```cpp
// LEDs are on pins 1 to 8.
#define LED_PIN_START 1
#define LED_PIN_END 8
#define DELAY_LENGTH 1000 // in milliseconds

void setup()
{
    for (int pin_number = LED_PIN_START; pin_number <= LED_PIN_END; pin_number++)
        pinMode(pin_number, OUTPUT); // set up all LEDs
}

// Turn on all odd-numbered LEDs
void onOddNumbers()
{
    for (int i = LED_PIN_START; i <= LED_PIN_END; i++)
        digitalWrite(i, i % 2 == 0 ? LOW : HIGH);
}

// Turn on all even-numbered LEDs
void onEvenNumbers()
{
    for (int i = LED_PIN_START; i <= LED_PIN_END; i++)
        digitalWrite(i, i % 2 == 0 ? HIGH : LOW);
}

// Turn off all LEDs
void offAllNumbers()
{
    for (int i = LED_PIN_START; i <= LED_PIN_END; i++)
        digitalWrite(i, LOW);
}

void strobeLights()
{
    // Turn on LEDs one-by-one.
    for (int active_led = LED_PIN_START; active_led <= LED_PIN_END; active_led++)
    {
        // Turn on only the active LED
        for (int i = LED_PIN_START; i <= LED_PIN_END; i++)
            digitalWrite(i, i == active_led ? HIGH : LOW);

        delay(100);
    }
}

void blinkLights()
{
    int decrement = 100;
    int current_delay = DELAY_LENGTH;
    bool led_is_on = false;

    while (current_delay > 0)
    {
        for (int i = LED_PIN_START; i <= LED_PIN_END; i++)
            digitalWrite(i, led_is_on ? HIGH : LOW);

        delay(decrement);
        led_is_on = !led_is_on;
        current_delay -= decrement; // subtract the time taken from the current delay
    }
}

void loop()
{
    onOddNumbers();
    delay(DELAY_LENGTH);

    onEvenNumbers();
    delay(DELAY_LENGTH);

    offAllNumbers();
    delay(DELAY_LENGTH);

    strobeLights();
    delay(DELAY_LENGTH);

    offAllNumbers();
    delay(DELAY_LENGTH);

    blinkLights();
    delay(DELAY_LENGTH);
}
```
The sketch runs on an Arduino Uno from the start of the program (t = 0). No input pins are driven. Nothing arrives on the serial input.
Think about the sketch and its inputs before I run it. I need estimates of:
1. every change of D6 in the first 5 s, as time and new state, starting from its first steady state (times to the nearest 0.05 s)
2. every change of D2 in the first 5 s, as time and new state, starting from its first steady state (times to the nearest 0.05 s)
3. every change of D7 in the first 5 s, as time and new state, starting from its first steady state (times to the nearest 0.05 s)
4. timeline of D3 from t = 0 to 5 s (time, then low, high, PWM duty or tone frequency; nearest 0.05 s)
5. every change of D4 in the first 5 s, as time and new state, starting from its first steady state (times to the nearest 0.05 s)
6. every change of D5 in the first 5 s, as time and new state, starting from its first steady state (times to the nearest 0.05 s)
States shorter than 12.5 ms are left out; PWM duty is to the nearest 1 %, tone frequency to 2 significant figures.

0 s low; 1 s high; 2 s low; 3.5 s high; 3.6 s low
0 s low; 1 s high; 2 s low; 3.1 s high; 3.2 s low
0 s high; 1 s low; 3.6 s high; 3.7 s low
0 s high; 1 s low; 3.2 s high; 3.3 s low
0 s low; 1 s high; 2 s low; 3.3 s high; 3.4 s low
0 s high; 1 s low; 3.4 s high; 3.5 s low
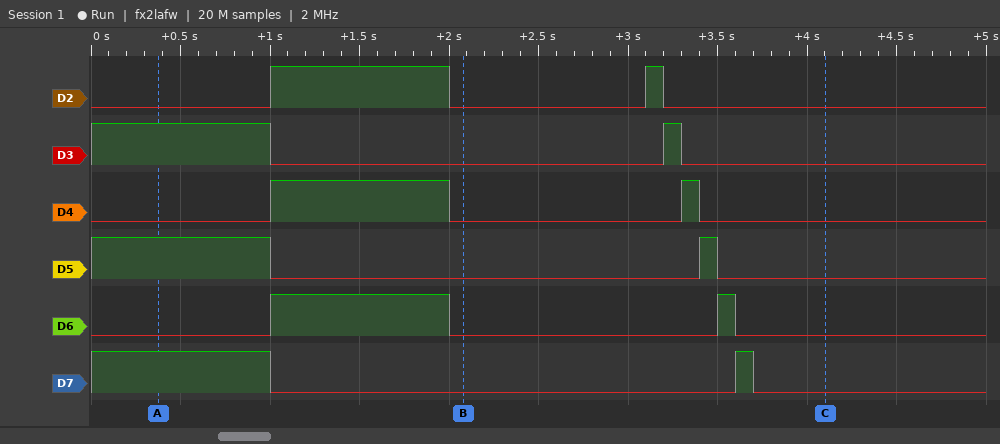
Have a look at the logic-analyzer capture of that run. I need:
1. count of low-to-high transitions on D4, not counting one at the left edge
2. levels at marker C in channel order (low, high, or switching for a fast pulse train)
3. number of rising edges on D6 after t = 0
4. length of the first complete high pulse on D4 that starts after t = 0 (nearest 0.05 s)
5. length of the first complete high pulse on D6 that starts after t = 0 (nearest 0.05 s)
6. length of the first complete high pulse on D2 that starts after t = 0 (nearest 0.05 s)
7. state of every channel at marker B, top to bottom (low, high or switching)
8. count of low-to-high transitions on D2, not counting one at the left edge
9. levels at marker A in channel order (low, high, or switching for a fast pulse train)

2
D2 low, D3 low, D4 low, D5 low, D6 low, D7 low
2
1.00 s
1.00 s
1.00 s
D2 low, D3 low, D4 low, D5 low, D6 low, D7 low
2
D2 low, D3 high, D4 low, D5 high, D6 low, D7 high
